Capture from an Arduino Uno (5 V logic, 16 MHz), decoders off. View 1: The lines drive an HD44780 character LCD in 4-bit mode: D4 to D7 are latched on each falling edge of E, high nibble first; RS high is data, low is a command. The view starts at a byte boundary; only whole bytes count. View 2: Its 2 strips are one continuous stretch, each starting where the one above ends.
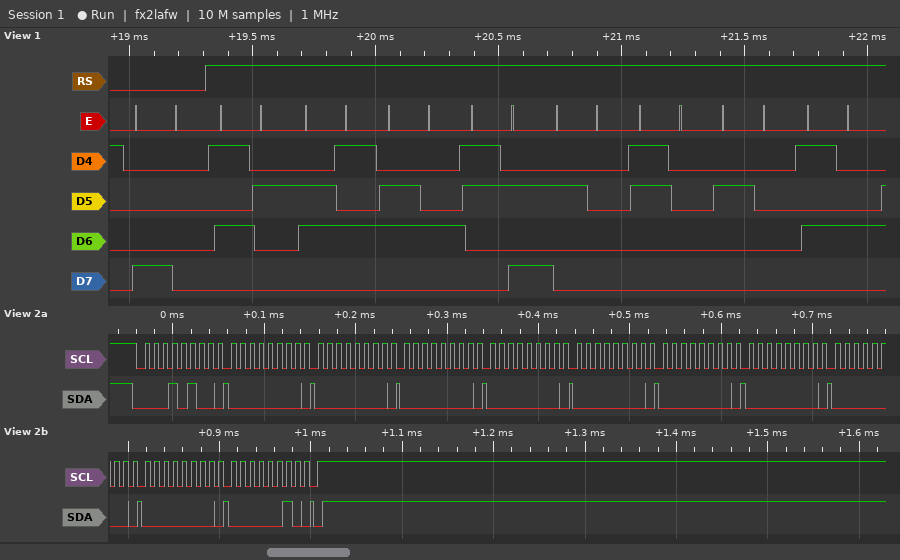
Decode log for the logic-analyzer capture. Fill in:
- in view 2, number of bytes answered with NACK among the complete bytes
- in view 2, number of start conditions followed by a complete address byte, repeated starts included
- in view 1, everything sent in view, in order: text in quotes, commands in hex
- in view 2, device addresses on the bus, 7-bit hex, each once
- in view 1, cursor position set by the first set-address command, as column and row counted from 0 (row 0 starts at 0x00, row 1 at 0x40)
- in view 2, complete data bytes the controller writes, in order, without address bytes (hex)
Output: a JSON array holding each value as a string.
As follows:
["0", "1", "0x80 \"Red: 0 T\"", "0x0A", "column 0, row 0", "00 00 00 00 00 00 00 00 00 02"]
